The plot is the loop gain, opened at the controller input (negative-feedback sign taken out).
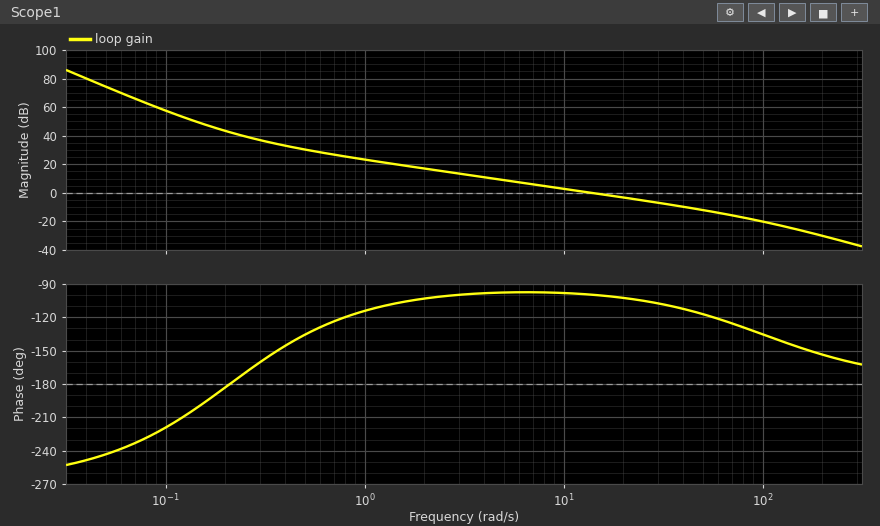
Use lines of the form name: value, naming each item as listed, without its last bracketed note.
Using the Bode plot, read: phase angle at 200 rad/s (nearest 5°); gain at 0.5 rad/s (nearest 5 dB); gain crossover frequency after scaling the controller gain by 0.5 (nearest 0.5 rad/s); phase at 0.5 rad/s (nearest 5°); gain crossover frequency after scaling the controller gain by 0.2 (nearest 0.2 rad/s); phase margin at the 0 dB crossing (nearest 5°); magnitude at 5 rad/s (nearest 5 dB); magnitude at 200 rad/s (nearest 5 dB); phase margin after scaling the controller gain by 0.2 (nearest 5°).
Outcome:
phase angle at 200 rad/s: -155°
gain at 0.5 rad/s: 30 dB
gain crossover frequency after scaling the controller gain by 0.5: 7.0 rad/s
phase at 0.5 rad/s: -135°
gain crossover frequency after scaling the controller gain by 0.2: 2.8 rad/s
phase margin at the 0 dB crossing: 80°
magnitude at 5 rad/s: 10 dB
magnitude at 200 rad/s: -30 dB
phase margin after scaling the controller gain by 0.2: 80°
